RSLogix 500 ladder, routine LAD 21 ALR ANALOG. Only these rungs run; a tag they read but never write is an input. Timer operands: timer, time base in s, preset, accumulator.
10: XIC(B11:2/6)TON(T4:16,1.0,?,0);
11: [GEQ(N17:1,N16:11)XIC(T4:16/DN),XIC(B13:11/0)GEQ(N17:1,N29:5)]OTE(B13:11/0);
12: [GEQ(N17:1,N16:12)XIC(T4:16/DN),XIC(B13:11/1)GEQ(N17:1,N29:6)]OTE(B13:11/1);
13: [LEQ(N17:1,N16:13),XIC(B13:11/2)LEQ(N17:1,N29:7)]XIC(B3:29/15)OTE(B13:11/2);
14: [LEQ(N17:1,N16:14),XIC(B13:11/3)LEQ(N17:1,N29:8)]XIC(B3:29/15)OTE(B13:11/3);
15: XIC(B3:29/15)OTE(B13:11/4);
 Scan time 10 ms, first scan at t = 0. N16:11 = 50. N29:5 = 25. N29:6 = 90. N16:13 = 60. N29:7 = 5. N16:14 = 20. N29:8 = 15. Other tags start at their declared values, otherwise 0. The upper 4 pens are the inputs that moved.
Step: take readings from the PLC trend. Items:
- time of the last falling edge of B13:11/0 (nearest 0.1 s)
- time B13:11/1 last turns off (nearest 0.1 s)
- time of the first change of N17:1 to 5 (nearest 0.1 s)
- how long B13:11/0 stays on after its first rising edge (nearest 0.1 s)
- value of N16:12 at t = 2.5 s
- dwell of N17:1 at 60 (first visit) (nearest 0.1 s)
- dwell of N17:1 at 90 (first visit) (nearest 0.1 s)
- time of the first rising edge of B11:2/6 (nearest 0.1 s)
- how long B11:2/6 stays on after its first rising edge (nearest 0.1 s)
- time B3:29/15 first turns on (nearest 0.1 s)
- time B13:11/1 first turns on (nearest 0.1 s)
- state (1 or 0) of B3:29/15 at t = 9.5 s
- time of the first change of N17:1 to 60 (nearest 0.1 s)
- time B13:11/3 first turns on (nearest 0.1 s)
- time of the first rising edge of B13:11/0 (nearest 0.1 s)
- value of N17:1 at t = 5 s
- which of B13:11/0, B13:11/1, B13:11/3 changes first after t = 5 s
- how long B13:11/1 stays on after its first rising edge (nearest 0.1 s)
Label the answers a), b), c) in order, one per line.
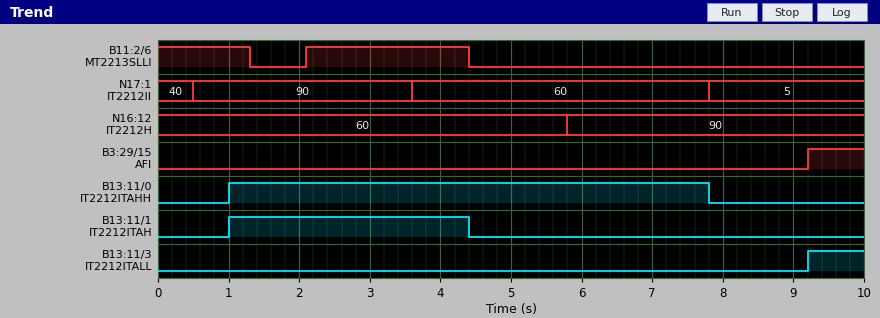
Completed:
a) 7.8 s
b) 4.4 s
c) 7.8 s
d) 6.8 s
e) 60
f) 4.2 s
g) 3.1 s
h) 2.1 s
i) 2.3 s
j) 9.2 s
k) 1.0 s
l) 1
m) 3.6 s
n) 9.2 s
o) 1.0 s
p) 60
q) B13:11/0
r) 3.4 s
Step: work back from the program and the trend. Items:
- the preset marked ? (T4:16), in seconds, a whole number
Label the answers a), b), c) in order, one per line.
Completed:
a) 1 s
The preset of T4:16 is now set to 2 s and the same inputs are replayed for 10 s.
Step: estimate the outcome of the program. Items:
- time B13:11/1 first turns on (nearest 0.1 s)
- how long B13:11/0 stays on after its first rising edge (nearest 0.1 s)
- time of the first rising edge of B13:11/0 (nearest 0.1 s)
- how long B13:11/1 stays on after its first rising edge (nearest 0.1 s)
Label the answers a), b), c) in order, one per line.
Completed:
a) 4.1 s
b) 3.7 s
c) 4.1 s
d) 0.3 s
